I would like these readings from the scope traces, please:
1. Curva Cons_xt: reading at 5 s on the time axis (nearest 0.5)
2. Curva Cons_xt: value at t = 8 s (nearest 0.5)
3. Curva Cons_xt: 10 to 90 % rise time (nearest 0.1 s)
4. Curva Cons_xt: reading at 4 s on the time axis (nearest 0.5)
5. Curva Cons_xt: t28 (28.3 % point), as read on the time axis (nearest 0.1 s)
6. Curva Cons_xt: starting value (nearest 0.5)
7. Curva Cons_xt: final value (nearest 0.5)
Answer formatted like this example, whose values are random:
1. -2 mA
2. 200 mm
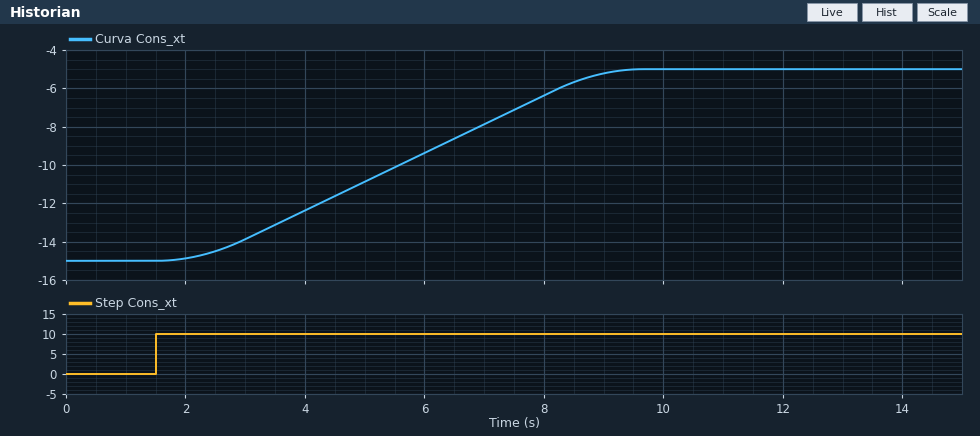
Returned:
1. -11.0
2. -6.5
3. 5.3 s
4. -12.5
5. 4.1 s
6. -15.0
7. -5.0
